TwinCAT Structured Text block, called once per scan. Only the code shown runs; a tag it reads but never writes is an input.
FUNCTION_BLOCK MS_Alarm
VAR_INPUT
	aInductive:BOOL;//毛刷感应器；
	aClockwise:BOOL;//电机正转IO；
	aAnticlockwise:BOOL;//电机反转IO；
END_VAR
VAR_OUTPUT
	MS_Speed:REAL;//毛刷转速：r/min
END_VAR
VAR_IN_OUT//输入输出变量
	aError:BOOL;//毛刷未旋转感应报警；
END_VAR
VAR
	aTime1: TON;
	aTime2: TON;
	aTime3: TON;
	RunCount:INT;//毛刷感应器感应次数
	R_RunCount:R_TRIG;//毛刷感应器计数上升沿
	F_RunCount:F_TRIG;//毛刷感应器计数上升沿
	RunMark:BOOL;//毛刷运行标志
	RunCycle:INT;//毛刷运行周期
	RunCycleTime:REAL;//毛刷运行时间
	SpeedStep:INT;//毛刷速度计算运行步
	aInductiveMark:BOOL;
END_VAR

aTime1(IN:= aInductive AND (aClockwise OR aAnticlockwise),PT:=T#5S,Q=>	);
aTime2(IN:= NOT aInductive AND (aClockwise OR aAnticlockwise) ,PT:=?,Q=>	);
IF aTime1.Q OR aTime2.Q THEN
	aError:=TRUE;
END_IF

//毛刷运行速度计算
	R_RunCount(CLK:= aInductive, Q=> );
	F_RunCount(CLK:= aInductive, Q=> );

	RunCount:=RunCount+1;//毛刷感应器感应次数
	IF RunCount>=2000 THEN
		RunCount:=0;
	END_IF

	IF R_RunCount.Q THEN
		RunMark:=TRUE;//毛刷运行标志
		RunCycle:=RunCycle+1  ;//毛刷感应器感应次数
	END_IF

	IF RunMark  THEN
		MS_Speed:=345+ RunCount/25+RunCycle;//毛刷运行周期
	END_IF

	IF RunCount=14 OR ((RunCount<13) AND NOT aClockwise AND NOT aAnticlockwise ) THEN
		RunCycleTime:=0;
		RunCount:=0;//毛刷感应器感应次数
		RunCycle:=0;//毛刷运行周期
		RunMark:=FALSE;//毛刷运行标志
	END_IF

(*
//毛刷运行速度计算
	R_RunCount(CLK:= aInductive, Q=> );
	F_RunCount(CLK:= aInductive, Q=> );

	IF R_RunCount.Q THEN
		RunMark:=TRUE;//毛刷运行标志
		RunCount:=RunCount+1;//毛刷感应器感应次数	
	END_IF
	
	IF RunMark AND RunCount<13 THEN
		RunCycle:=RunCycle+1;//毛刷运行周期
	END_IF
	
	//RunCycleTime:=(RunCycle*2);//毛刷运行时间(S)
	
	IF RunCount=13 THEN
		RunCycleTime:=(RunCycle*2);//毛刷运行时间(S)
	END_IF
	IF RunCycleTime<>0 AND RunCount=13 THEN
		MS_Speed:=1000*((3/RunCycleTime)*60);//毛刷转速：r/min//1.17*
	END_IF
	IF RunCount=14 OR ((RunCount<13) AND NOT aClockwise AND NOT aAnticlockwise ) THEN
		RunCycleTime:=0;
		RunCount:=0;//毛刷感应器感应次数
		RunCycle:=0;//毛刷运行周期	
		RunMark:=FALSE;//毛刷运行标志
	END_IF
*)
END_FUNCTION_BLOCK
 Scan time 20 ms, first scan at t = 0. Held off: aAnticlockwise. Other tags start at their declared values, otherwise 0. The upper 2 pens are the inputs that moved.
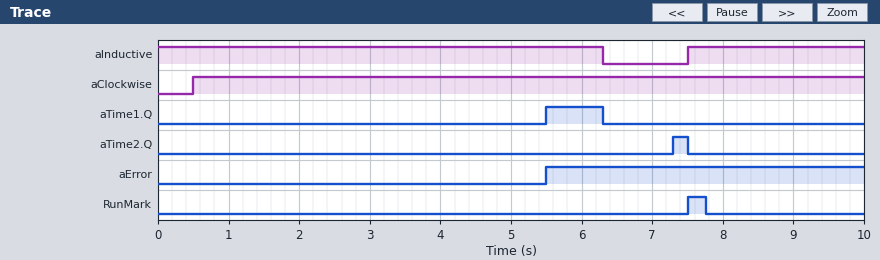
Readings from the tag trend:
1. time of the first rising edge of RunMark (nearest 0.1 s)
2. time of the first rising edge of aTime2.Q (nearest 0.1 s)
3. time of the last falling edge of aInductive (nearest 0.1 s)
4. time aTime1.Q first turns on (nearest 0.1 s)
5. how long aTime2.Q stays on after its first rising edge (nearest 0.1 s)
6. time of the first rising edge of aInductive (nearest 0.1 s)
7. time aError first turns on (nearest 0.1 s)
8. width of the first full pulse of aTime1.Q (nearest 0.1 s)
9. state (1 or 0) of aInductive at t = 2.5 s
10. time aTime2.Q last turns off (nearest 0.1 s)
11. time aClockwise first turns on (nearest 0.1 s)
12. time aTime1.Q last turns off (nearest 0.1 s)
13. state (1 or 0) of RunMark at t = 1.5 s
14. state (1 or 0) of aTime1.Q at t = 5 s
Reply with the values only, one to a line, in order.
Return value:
7.5 s
7.3 s
6.3 s
5.5 s
0.2 s
7.5 s
5.5 s
0.8 s
1
7.5 s
0.5 s
6.3 s
0
0
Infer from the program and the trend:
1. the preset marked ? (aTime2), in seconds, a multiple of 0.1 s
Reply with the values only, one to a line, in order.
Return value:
1.0 s
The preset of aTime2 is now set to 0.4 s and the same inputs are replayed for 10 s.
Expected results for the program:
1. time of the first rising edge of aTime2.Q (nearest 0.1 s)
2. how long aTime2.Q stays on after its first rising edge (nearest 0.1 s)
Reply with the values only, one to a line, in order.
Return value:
6.7 s
0.8 s
